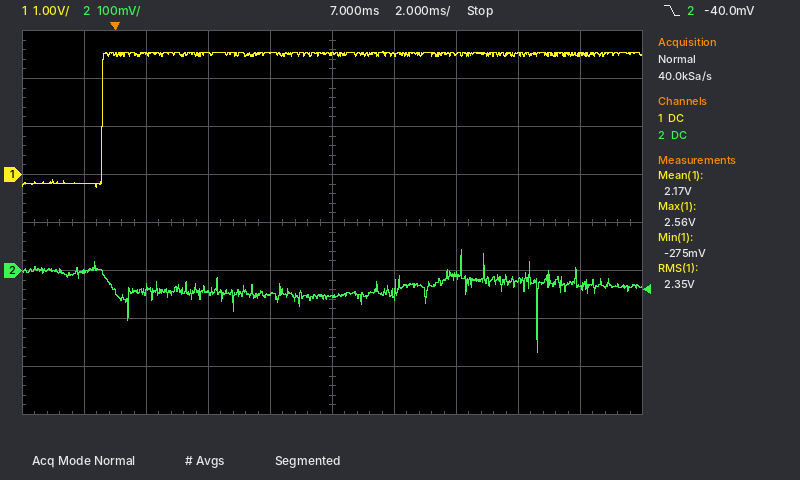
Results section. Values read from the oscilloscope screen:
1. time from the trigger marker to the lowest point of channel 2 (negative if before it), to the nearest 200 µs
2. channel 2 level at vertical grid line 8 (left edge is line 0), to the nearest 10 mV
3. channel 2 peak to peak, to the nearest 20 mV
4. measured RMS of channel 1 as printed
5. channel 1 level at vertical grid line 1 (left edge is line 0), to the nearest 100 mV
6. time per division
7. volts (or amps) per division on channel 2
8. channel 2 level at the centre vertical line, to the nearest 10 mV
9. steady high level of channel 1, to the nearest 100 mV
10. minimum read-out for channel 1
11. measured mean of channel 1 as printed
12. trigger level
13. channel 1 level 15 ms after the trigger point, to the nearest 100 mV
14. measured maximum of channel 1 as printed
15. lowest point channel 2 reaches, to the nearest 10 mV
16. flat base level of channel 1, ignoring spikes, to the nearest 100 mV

+13.6 ms
-20 mV
220 mV
2.35 V
-200 mV
2 ms
100 mV
-50 mV
2.5 V
-275 mV
2.17 V
-40.0 mV
2.5 V
2.56 V
-170 mV
-200 mV
